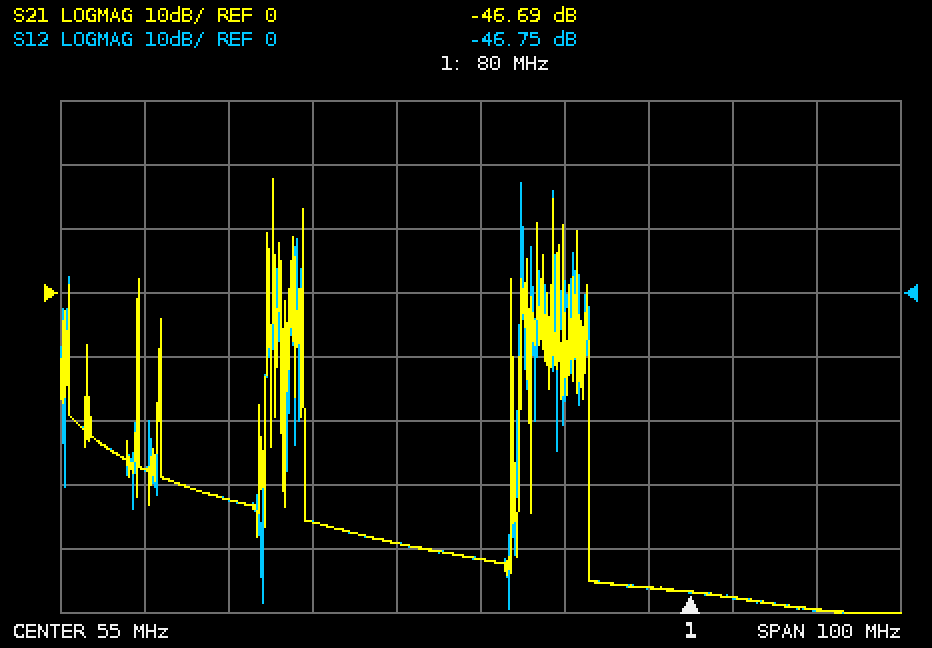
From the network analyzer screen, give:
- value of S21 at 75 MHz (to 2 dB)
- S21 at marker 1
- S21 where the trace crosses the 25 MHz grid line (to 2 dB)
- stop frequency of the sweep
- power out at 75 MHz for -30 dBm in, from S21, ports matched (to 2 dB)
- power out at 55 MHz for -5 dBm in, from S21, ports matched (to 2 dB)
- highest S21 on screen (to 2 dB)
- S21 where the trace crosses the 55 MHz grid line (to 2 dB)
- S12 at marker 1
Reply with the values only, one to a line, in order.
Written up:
-46 dB
-46.69 dB
-32 dB
105 MHz
-76 dBm
-46 dBm
18 dB
-42 dB
-46.75 dB
